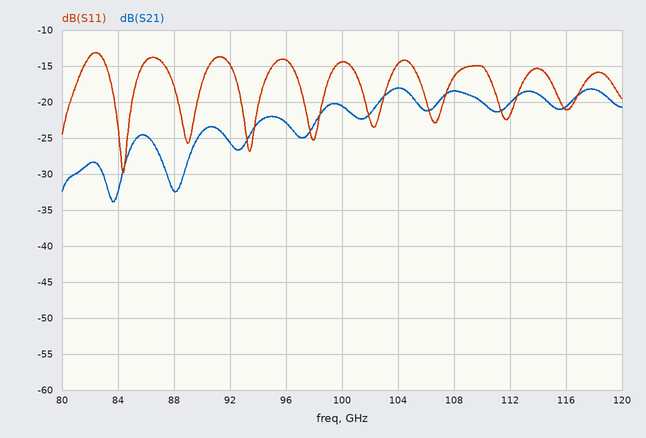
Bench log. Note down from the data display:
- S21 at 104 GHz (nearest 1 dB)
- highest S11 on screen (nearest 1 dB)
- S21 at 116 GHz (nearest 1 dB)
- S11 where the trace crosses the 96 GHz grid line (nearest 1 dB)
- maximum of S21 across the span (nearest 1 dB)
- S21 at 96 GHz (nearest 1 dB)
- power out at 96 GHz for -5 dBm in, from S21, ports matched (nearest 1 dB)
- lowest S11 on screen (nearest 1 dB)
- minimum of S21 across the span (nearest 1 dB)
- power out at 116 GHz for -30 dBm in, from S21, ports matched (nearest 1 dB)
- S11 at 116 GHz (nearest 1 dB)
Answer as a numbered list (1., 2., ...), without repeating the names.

1. -18 dB
2. -13 dB
3. -21 dB
4. -14 dB
5. -18 dB
6. -23 dB
7. -28 dBm
8. -30 dB
9. -34 dB
10. -51 dBm
11. -21 dB
